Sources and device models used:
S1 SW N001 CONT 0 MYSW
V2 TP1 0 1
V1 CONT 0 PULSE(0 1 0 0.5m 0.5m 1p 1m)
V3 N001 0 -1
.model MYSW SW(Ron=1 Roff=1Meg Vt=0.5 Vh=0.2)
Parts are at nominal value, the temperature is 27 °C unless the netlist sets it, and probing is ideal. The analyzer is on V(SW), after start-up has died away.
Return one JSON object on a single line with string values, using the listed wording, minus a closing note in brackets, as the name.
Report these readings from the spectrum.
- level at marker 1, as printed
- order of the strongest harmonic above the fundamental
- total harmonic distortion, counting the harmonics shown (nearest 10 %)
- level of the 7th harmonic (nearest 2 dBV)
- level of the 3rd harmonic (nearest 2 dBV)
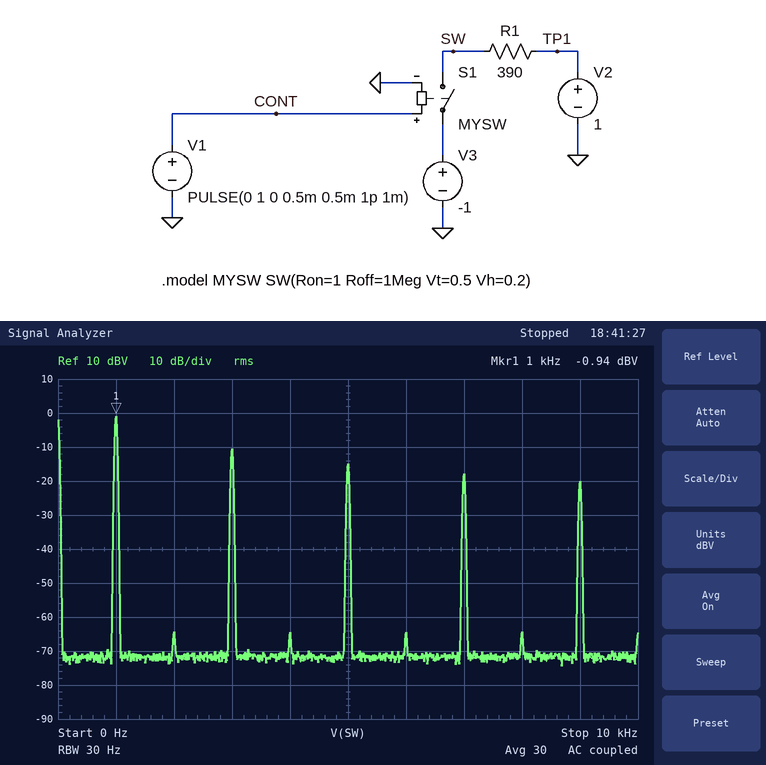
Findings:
{"level at marker 1, as printed": "-0.94 dBV", "order of the strongest harmonic above the fundamental": "3", "total harmonic distortion, counting the harmonics shown": "40 %", "level of the 7th harmonic": "-18 dBV", "level of the 3rd harmonic": "-10 dBV"}
